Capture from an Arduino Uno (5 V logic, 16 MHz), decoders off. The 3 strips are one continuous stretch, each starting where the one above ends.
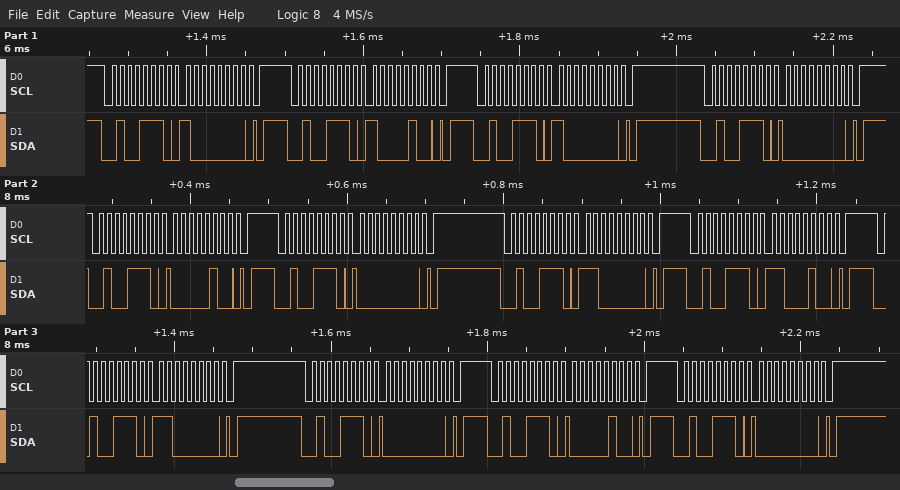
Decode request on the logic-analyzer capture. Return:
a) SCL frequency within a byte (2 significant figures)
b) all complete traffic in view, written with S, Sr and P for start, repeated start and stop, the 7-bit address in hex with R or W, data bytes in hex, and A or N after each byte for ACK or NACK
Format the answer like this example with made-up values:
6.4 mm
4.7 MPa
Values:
100 kHz
S 27W A 80 A P S 27W A 84 A P S 27W A 80 A P S 27W A 00 A P S 27W A 04 A P S 27W A 00 A P S 27W A C0 A P S 27W A C4 A P S 27W A C0 A P S 27W A 00 A P S 27W A 04 A P S 27W A 00 A P
